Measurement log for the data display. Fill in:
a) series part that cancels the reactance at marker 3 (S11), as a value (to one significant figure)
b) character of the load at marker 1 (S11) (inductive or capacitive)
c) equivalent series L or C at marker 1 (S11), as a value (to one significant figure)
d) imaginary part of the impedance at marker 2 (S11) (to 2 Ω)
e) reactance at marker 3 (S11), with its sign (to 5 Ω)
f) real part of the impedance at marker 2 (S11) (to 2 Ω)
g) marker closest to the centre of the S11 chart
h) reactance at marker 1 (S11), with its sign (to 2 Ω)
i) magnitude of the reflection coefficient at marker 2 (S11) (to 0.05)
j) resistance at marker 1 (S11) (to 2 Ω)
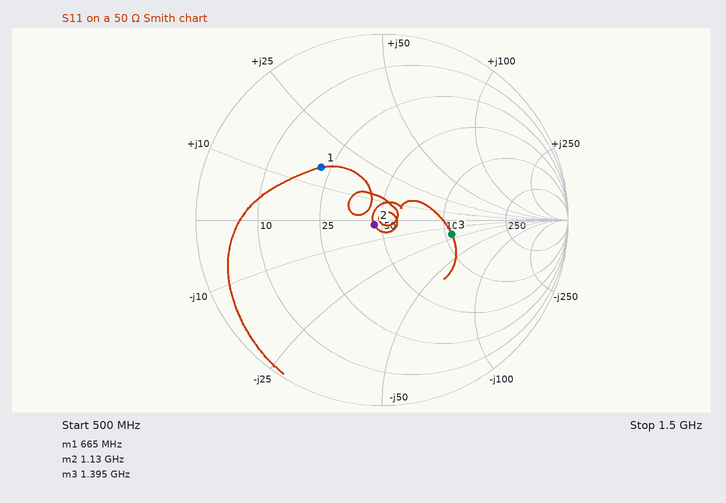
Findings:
2 nH
inductive
4 nH
-2 Ω
-20 Ω
46 Ω
marker 2
+16 Ω
0.05
22 Ω
